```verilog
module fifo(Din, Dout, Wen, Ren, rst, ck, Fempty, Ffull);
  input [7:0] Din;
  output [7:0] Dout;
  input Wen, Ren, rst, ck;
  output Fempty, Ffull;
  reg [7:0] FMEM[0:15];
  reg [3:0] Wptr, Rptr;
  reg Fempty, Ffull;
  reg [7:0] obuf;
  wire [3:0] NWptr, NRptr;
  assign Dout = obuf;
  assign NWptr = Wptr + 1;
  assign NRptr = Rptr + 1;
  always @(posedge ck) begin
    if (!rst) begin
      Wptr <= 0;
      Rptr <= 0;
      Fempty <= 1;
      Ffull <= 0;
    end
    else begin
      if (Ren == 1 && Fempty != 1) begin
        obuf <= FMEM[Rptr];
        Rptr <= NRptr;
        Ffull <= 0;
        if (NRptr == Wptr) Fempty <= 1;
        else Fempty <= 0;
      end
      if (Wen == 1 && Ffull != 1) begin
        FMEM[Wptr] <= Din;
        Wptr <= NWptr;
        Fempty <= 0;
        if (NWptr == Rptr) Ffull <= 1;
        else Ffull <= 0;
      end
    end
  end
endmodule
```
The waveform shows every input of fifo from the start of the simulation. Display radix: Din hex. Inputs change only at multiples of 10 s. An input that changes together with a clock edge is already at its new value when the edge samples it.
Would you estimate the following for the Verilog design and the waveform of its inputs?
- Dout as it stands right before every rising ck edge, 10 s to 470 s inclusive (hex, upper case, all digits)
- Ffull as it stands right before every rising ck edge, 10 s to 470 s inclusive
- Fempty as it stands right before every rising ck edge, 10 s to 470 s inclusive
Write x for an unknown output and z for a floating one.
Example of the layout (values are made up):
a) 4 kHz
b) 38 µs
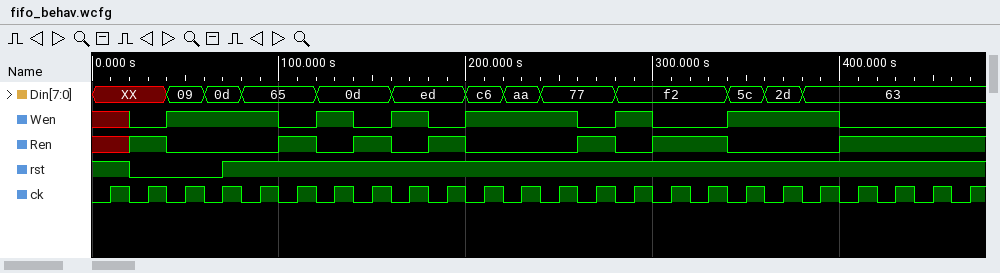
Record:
a) x, x, x, x, x, x, 0D, 0D, 65, 65, 0D, 0D, 0D, 0D, ED, ED, C6, AA, AA, AA, AA, 77, F2, 5C
b) x x 0 0 0 0 0 0 0 0 0 0 0 0 0 0 0 0 0 0 0 0 0 0
c) x x 1 1 0 0 0 0 0 0 0 0 0 0 0 0 0 0 0 0 0 0 0 0
